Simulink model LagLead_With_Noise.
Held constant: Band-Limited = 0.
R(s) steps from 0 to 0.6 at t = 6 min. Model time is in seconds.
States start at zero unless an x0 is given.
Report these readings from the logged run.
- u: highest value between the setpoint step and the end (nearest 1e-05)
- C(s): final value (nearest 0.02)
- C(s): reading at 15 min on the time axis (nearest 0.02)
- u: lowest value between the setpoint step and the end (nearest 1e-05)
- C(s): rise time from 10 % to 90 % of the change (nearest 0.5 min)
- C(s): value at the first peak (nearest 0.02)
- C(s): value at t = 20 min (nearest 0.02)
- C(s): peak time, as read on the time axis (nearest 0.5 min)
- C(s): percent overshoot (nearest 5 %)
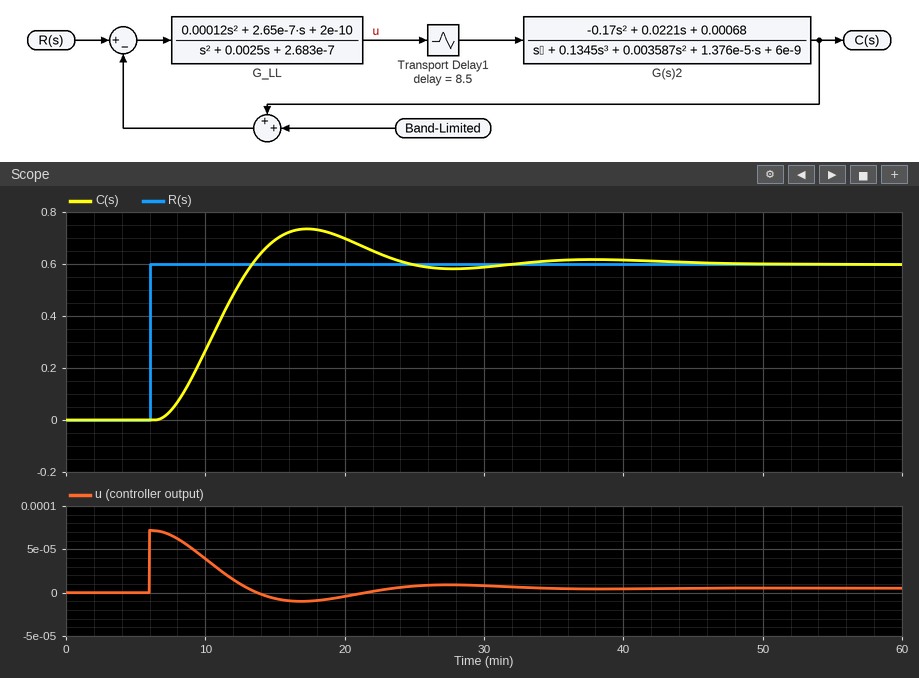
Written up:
0.00007
0.60
0.70
-0.00001
4.5 min
0.74
0.70
17.5 min
25 %
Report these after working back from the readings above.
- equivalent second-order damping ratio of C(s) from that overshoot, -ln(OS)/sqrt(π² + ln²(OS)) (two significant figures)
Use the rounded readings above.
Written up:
0.40
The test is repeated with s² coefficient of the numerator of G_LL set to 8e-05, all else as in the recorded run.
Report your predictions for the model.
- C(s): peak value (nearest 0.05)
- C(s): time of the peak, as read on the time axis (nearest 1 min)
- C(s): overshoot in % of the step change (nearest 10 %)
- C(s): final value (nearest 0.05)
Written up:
0.80
20 min
30 %
0.60
